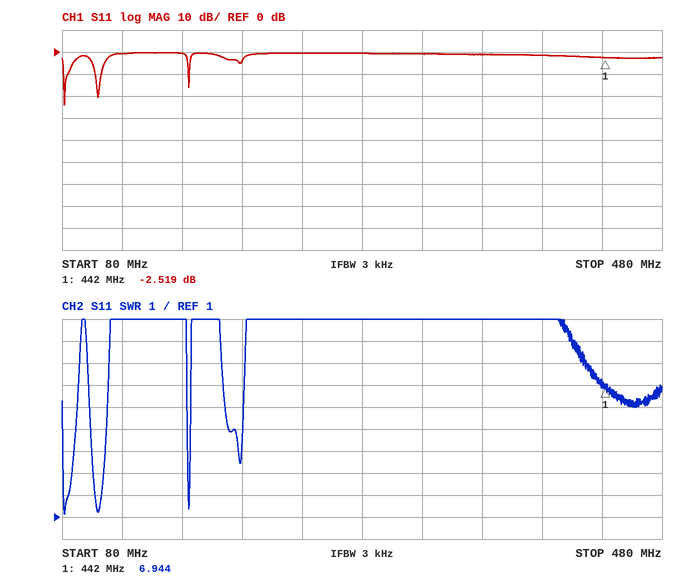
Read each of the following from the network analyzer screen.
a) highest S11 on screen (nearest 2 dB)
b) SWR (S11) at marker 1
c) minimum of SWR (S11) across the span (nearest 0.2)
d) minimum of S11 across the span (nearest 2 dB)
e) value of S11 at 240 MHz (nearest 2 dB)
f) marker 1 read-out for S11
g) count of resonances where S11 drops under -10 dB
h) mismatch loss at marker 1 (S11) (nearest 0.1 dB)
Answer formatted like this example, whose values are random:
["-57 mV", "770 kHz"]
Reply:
["0 dB", "6.944", "1.2", "-24 dB", "0 dB", "-2.519 dB", "3", "3.6 dB"]
